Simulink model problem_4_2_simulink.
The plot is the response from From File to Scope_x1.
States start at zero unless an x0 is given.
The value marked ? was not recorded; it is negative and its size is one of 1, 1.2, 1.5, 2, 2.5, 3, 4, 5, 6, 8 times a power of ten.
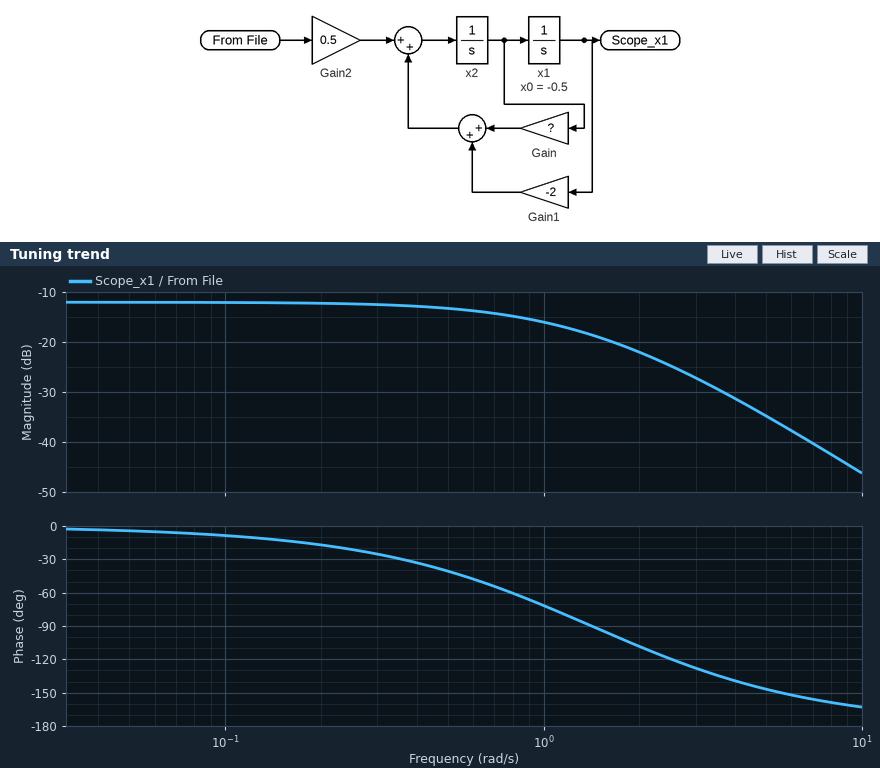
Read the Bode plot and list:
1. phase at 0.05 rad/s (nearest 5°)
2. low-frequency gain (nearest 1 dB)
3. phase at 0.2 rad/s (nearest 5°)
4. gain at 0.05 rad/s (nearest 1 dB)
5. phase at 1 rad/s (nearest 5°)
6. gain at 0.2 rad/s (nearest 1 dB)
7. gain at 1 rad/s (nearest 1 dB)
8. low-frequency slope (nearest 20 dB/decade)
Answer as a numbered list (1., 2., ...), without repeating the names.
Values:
1. -5°
2. -12 dB
3. -15°
4. -12 dB
5. -70°
6. -12 dB
7. -16 dB
8. 0 dB/decade
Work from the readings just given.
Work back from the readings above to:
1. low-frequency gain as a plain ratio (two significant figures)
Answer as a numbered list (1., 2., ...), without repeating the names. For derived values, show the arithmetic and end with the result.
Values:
1. 10^(-12 / 20) = 0.25
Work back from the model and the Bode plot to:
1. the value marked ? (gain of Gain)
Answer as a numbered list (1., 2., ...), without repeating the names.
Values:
1. -3
